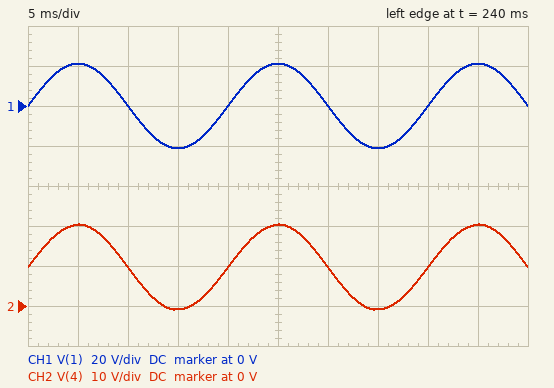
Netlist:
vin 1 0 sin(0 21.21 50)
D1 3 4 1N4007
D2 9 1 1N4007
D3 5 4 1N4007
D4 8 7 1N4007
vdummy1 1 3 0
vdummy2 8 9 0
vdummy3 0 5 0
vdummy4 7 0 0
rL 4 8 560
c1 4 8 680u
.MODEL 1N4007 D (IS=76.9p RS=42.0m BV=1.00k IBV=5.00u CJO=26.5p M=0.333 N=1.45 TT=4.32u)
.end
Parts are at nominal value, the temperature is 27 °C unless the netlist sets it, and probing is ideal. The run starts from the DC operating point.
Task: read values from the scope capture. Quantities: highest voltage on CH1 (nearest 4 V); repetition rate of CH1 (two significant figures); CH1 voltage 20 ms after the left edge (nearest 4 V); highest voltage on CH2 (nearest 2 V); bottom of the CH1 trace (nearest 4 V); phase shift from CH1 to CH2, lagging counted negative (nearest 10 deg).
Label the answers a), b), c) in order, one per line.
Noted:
a) 20 V
b) 50 Hz
c) 0 V
d) 20 V
e) -20 V
f) 0 deg
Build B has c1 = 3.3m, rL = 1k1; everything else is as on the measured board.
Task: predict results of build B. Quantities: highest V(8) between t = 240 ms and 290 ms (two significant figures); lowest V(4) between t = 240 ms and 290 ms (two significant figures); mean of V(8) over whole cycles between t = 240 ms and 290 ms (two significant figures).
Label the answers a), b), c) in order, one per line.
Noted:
a) 850 mV
b) -850 mV
c) -9.8 V
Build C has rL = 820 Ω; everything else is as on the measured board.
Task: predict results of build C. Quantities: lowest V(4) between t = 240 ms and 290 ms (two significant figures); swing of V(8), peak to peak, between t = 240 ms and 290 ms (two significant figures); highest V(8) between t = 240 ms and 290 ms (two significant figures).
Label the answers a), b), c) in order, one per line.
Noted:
a) -860 mV
b) 21 V
c) 860 mV
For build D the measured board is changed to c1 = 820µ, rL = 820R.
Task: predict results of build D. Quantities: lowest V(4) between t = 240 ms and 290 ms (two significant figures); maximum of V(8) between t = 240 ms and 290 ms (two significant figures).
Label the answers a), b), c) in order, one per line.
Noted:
a) -860 mV
b) 860 mV
